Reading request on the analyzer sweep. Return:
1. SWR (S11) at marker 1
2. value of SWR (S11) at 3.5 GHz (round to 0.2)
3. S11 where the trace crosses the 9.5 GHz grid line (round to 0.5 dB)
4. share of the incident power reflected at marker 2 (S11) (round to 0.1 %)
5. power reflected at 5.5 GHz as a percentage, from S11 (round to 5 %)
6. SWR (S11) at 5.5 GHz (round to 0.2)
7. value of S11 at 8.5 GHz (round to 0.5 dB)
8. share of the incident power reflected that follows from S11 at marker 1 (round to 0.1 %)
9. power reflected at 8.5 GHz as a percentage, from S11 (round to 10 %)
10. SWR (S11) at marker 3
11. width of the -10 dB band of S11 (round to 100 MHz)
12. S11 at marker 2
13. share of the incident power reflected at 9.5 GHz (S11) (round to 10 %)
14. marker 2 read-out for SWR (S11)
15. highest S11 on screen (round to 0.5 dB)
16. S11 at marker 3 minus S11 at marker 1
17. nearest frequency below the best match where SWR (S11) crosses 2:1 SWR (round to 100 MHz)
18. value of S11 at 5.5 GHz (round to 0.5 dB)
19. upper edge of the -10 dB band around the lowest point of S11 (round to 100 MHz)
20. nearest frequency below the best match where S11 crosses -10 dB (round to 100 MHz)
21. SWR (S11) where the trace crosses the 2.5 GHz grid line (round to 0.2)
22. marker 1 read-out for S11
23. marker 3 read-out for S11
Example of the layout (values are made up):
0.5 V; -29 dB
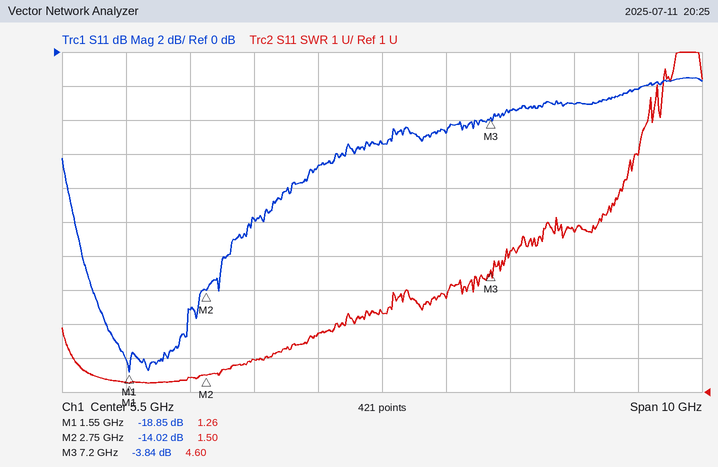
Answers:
1.26; 2.0; -2.0 dB; 4.0 %; 30 %; 3.4; -3.0 dB; 1.3 %; 50 %; 4.60; 2.8 GHz; -14.02 dB; 60 %; 1.50; -1.5 dB; 15.01 dB; 700 MHz; -5.5 dB; 3.5 GHz; 700 MHz; 1.4; -18.85 dB; -3.84 dB
